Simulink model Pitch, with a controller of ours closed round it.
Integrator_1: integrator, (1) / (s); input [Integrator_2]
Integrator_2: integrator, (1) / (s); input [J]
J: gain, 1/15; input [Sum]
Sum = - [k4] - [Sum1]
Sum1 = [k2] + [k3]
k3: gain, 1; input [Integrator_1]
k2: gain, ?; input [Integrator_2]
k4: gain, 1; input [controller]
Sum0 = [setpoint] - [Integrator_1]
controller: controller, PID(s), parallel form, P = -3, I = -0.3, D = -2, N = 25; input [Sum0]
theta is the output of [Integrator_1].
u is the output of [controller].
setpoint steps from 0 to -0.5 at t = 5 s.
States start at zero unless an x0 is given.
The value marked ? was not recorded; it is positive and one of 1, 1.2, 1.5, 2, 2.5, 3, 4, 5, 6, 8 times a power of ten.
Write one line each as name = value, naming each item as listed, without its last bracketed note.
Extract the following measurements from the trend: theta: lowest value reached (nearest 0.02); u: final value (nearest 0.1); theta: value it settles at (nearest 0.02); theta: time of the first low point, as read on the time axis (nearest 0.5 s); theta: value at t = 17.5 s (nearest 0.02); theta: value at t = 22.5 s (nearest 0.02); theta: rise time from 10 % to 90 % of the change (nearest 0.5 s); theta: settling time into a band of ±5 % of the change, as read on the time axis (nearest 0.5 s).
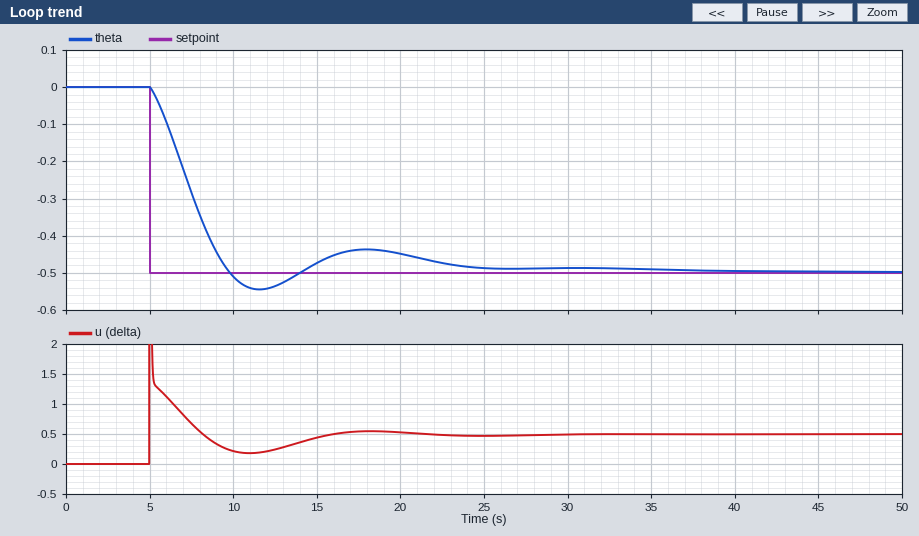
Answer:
theta: lowest value reached = -0.54
u: final value = 0.5
theta: value it settles at = -0.50
theta: time of the first low point, as read on the time axis = 11.5 s
theta: value at t = 17.5 s = -0.44
theta: value at t = 22.5 s = -0.48
theta: rise time from 10 % to 90 % of the change = 3.5 s
theta: settling time into a band of ±5 % of the change, as read on the time axis = 22.5 s
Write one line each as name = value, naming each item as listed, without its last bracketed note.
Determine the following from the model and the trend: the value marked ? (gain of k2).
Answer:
the value marked ? = 5
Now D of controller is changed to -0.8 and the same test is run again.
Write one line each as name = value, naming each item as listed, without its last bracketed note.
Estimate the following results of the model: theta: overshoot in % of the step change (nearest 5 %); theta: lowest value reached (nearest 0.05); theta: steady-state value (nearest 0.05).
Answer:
theta: overshoot in % of the step change = 15 %
theta: lowest value reached = -0.60
theta: steady-state value = -0.50
